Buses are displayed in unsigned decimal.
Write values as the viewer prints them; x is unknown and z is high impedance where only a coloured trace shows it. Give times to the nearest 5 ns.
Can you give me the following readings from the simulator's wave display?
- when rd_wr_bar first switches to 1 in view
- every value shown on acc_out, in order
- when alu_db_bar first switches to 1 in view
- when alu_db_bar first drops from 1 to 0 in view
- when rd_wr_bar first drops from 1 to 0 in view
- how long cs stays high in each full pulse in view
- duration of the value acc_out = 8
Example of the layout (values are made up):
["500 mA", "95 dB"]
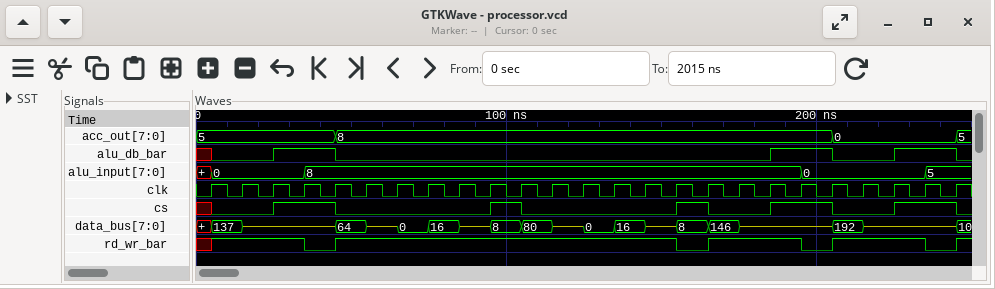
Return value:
["5 ns", "5, 8, 0, 5", "25 ns", "45 ns", "35 ns", "20 ns, 10 ns, 10 ns, 20 ns, 20 ns", "160 ns"]
